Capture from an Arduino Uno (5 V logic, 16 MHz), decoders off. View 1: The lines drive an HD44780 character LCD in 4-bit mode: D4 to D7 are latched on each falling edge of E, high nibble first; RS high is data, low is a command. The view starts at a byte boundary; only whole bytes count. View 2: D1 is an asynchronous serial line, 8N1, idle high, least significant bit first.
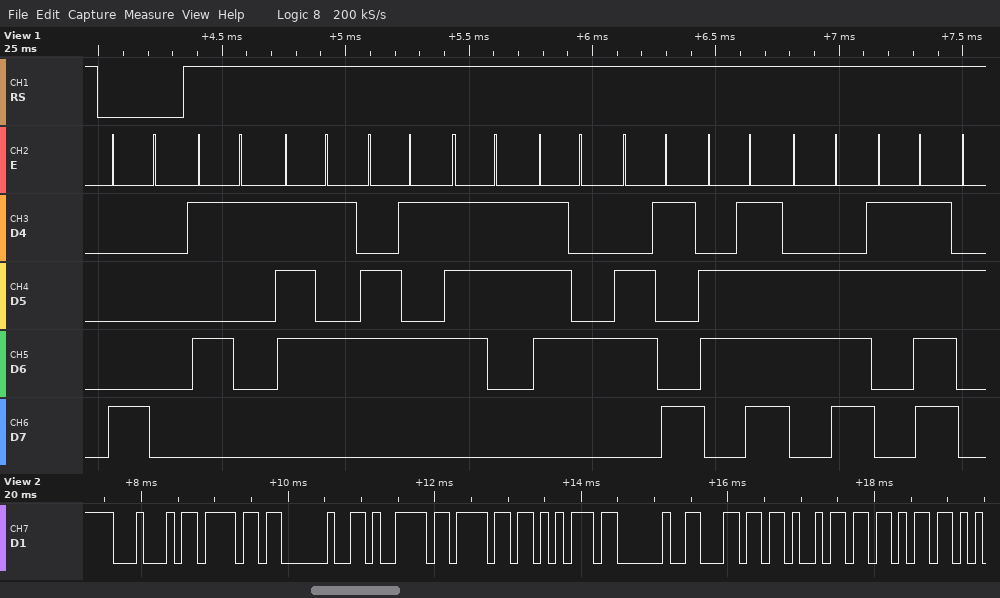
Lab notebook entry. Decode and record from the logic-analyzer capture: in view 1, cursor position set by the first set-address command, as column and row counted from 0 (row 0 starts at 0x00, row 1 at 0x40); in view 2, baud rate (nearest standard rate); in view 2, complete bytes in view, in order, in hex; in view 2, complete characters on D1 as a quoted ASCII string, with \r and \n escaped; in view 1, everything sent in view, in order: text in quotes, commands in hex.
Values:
column 0, row 0
9600 baud
44 6F 20 79 6F 75 20 6C 69 6B
"Do you lik"
0x80 "Question?"
